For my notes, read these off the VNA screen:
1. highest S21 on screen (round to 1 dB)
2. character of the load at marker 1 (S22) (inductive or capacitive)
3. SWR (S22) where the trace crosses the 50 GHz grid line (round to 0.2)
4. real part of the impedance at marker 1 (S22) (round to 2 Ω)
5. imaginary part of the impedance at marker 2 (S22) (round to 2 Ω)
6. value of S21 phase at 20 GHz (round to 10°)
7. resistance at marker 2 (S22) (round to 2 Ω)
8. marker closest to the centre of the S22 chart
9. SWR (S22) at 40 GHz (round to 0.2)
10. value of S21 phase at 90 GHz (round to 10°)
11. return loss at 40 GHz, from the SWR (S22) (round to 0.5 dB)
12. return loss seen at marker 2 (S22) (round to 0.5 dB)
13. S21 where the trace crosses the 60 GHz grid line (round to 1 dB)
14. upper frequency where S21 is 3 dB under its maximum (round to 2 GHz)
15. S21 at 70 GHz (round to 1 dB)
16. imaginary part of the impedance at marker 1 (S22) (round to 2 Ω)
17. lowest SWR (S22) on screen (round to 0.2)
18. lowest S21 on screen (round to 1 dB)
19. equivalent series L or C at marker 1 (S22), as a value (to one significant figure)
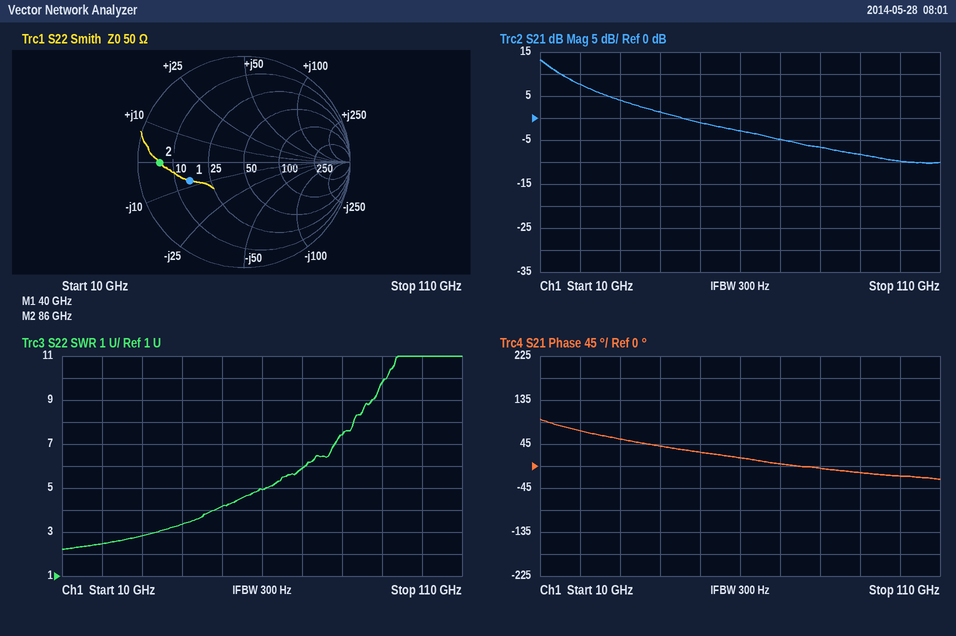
13 dB
capacitive
4.2
16 Ω
0 Ω
70°
6 Ω
marker 1
3.4
-10°
5.5 dB
2.0 dB
-3 dB
14 GHz
-5 dB
-8 Ω
2.2
-10 dB
500 fF
